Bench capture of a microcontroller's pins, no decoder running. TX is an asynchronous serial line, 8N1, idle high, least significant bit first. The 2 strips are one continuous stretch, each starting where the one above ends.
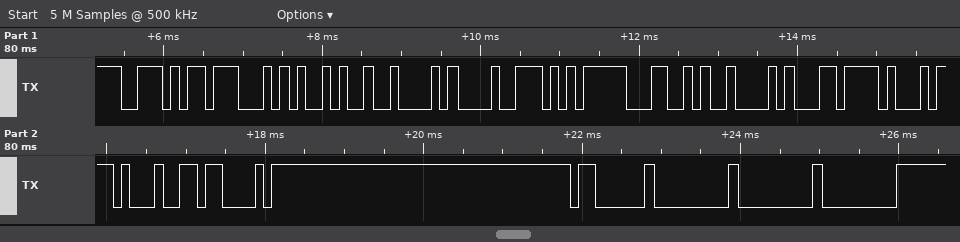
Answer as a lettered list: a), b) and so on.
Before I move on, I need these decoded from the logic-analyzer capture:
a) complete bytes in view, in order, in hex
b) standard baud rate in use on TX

a) 0xAE 0x47 0x29 0x42 0xC8 0xF5 0x4C 0x42 0xEC 0xD1 0x91 0x43 0x03 0x00 0x00 0x00
b) 9600 baud
